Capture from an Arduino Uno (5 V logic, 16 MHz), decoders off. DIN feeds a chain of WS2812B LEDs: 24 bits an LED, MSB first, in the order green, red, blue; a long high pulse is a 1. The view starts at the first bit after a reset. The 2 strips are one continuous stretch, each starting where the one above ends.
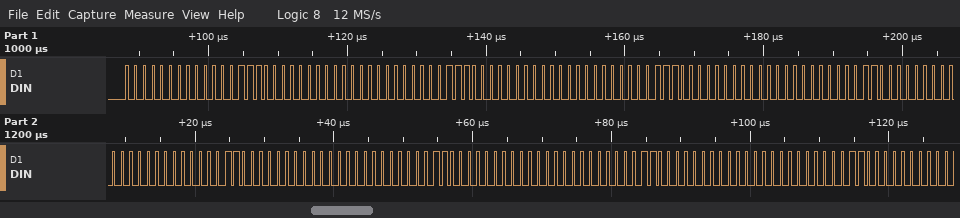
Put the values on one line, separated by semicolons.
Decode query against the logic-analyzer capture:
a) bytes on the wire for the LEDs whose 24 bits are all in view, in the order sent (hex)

00 07 00 00 07 00 00 07 00 00 06 00 00 06 00 00 06 00 00 06 00 00 06 00
